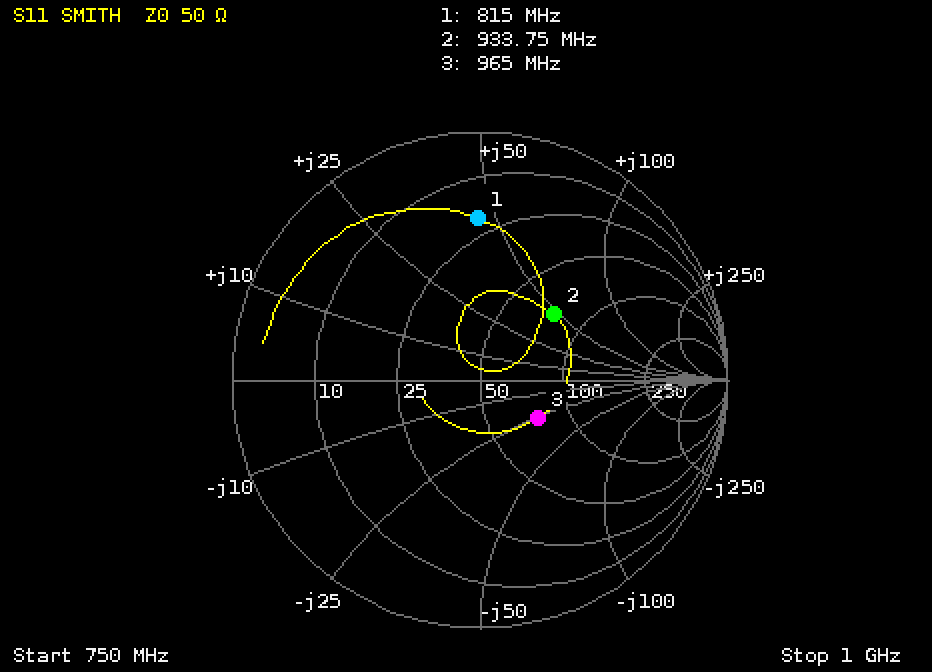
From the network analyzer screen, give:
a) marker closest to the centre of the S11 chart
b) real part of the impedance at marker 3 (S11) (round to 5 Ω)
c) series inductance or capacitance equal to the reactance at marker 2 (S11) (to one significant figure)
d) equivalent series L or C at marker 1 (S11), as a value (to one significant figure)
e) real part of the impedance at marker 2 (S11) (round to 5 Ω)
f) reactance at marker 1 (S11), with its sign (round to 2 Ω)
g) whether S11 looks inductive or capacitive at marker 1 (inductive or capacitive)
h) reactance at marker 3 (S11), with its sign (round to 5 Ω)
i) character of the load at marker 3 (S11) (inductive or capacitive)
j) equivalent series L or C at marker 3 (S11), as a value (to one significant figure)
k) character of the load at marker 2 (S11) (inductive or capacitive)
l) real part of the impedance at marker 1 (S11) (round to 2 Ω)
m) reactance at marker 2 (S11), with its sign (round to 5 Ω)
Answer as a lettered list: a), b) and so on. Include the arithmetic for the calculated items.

a) marker 3
b) 75 Ω
c) L = 45 Ω/(2π × 933.75 MHz) ≈ 8 nH
d) L = 46 Ω/(2π × 815 MHz) ≈ 9 nH
e) 75 Ω
f) +46 Ω
g) inductive
h) -25 Ω
i) capacitive
j) C = 1/(2π × 965 MHz × 25 Ω) ≈ 7 pF
k) inductive
l) 20 Ω
m) +45 Ω
